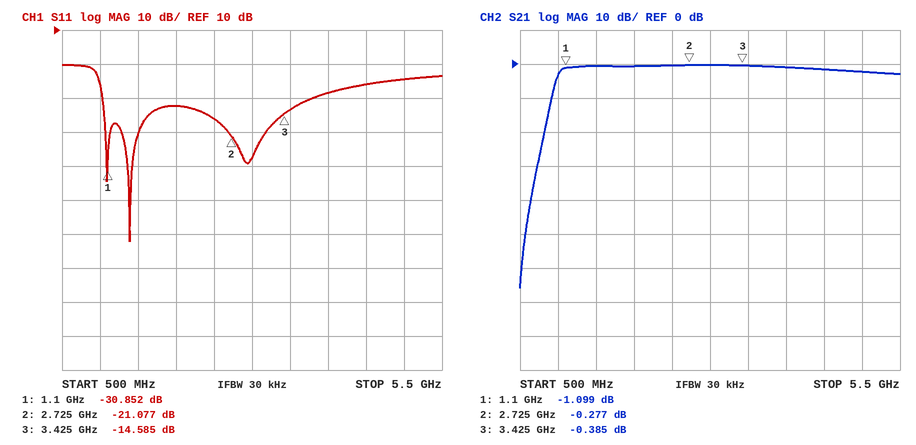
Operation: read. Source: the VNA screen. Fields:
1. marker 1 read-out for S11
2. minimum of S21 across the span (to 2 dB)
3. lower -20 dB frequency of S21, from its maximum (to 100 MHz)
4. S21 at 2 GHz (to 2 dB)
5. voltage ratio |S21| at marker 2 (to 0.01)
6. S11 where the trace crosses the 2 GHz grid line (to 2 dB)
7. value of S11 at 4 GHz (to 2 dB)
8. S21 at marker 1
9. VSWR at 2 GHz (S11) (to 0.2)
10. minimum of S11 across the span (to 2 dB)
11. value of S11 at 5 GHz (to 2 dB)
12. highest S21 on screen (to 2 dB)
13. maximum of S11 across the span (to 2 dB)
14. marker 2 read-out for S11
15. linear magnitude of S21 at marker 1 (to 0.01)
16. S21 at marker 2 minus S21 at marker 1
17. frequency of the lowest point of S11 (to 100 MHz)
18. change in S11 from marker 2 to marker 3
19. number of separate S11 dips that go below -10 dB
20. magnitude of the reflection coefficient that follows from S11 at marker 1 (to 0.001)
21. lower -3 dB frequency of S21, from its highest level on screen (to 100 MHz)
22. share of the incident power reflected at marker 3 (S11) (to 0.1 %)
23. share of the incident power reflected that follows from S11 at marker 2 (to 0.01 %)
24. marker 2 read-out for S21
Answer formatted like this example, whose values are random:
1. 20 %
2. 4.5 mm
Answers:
1. -30.852 dB
2. -66 dB
3. 800 MHz
4. 0 dB
5. 0.97
6. -12 dB
7. -8 dB
8. -1.099 dB
9. 1.6
10. -52 dB
11. -4 dB
12. 0 dB
13. 0 dB
14. -21.077 dB
15. 0.88
16. 0.822 dB
17. 1.4 GHz
18. 6.492 dB
19. 3
20. 0.029
21. 1.0 GHz
22. 3.5 %
23. 0.78 %
24. -0.277 dB
